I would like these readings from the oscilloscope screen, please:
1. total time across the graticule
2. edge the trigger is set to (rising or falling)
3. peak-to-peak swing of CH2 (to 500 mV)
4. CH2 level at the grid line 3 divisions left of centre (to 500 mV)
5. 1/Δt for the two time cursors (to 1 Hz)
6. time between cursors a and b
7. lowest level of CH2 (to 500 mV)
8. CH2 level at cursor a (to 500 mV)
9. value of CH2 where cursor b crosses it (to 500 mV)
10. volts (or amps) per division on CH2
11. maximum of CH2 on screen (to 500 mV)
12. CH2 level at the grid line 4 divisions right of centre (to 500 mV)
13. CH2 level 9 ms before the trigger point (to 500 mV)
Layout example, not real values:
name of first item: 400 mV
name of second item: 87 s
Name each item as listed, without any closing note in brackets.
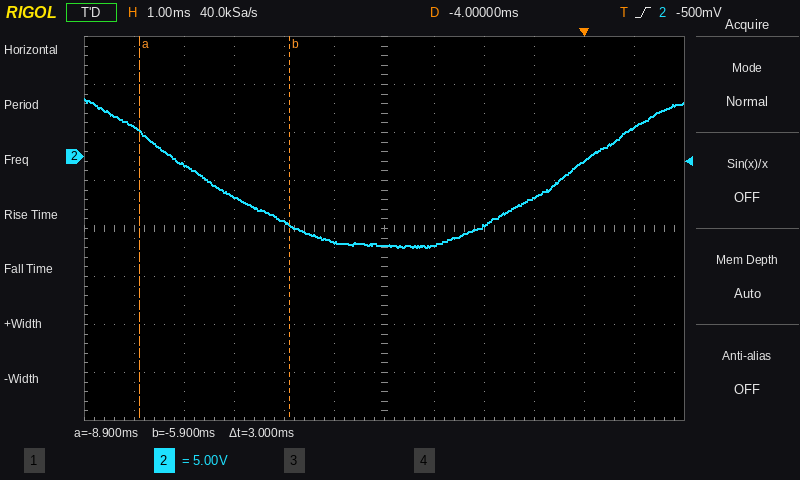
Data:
total time across the graticule: 12 ms
edge the trigger is set to: rising
peak-to-peak swing of CH2: 15.5 V
CH2 level at the grid line 3 divisions left of centre: -4.0 V
1/Δt for the two time cursors: 333 Hz
time between cursors a and b: 3 ms
lowest level of CH2: -9.5 V
CH2 level at cursor a: 2.5 V
value of CH2 where cursor b crosses it: -7.0 V
volts (or amps) per division on CH2: 5 V
maximum of CH2 on screen: 6.0 V
CH2 level at the grid line 4 divisions right of centre: -500 mV
CH2 level 9 ms before the trigger point: 3.0 V
